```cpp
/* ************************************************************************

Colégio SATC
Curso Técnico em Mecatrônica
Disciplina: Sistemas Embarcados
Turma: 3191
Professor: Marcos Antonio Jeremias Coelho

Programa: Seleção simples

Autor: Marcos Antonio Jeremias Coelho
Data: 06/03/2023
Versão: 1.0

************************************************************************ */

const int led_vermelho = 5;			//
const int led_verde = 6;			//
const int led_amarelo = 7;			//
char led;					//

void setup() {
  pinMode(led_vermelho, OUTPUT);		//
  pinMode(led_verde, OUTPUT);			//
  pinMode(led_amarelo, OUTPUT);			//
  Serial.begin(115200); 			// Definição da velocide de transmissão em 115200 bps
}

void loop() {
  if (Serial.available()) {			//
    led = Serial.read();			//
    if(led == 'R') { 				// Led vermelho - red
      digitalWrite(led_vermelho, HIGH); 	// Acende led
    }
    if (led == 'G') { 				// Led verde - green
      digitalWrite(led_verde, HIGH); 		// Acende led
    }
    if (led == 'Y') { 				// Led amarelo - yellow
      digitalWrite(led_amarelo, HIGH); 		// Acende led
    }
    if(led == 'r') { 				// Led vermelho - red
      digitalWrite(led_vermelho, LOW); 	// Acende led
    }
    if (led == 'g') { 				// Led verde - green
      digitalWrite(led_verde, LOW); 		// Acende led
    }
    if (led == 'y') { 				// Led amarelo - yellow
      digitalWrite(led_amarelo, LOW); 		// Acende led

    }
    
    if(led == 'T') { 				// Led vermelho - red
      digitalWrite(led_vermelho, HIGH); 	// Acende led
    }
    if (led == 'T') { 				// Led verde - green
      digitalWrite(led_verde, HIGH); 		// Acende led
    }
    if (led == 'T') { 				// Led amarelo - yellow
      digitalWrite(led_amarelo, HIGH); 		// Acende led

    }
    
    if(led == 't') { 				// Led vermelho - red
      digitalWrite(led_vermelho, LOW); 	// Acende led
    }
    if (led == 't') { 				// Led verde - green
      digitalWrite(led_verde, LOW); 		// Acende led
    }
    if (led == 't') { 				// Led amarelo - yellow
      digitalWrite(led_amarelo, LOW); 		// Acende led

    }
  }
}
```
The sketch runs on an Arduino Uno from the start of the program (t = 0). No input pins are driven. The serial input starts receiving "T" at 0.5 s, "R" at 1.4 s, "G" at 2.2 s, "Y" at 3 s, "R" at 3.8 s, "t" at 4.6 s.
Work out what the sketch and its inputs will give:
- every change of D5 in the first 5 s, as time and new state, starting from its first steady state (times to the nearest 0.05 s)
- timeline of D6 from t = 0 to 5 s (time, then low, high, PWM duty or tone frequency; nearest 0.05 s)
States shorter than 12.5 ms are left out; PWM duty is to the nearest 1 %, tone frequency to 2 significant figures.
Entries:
0 s low; 0.5 s high; 4.6 s low
0 s low; 0.5 s high; 4.6 s low
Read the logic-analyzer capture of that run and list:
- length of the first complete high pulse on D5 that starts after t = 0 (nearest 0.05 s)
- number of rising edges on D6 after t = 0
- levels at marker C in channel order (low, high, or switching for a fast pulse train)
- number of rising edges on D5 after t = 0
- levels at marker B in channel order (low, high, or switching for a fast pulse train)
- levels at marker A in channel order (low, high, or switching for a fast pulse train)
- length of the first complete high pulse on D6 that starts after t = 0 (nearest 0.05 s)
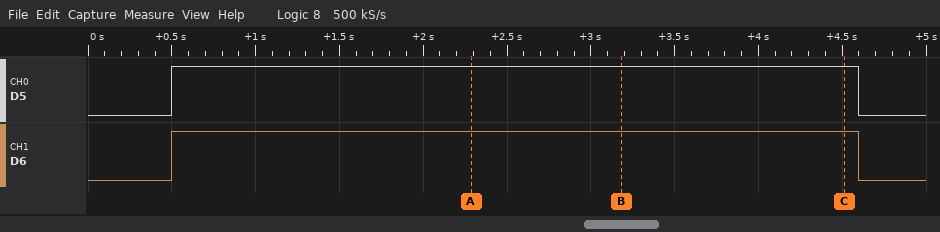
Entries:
4.10 s
1
D5 high, D6 high
1
D5 high, D6 high
D5 high, D6 high
4.10 s
